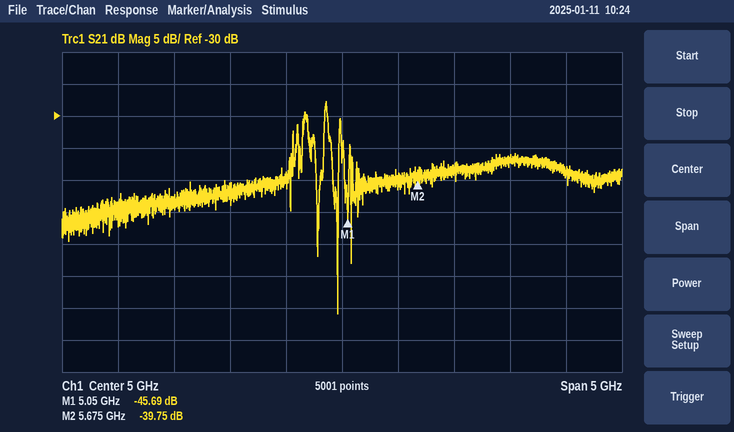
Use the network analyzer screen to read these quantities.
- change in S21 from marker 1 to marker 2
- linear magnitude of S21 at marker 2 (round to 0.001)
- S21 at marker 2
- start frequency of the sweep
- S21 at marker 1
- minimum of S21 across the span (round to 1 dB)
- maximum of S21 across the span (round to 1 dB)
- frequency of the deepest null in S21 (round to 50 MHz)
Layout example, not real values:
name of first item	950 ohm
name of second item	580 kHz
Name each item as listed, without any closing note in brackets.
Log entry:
change in S21 from marker 1 to marker 2	5.94 dB
linear magnitude of S21 at marker 2	0.010
S21 at marker 2	-39.75 dB
start frequency of the sweep	2.5 GHz
S21 at marker 1	-45.69 dB
minimum of S21 across the span	-61 dB
maximum of S21 across the span	-28 dB
frequency of the deepest null in S21	4.95 GHz
